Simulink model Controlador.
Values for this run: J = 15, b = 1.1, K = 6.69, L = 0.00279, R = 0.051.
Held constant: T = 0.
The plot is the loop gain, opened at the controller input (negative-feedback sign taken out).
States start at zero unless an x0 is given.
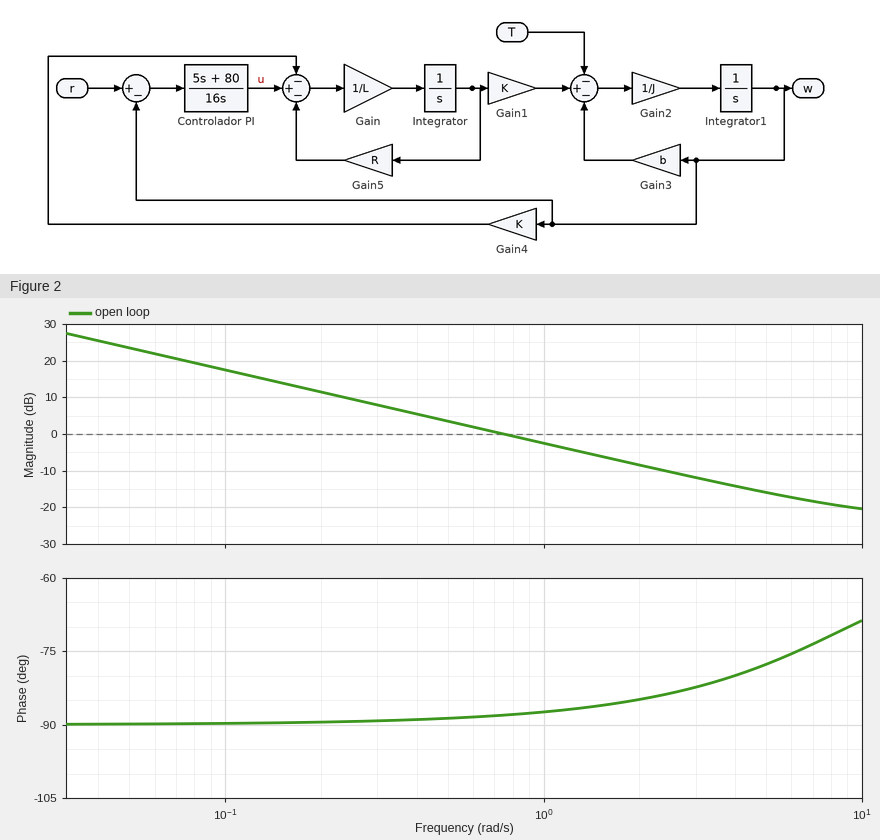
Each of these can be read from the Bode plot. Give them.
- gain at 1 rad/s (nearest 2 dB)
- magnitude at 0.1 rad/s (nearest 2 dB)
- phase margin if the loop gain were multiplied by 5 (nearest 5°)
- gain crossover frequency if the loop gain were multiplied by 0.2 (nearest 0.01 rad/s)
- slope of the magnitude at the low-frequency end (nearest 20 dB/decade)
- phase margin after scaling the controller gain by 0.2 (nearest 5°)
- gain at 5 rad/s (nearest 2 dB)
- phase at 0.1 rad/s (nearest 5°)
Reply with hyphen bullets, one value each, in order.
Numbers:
- -2 dB
- 18 dB
- 100°
- 0.15 rad/s
- -20 dB/decade
- 90°
- -16 dB
- -90°
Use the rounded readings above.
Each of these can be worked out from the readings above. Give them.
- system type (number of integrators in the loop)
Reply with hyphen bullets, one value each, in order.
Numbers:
- 1
